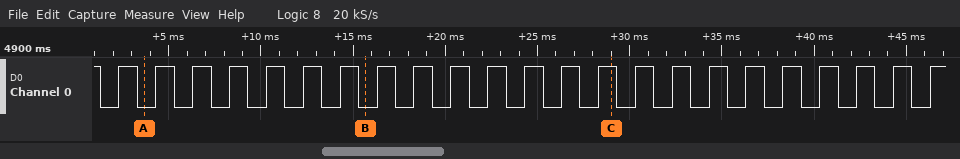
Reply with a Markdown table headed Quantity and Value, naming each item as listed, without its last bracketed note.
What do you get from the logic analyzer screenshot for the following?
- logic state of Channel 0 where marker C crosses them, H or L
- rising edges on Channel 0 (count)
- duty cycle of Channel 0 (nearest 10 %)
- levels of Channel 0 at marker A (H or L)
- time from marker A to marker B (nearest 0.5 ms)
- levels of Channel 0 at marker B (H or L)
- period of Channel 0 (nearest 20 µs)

| Quantity | Value |
|---|---|
| logic state of Channel 0 where marker C crosses them, H or L | Channel 0=H |
| rising edges on Channel 0 | 23 |
| duty cycle of Channel 0 | 50 % |
| levels of Channel 0 at marker A | Channel 0=L |
| time from marker A to marker B | 12 ms |
| levels of Channel 0 at marker B | Channel 0=L |
| period of Channel 0 | 2000 µs |
